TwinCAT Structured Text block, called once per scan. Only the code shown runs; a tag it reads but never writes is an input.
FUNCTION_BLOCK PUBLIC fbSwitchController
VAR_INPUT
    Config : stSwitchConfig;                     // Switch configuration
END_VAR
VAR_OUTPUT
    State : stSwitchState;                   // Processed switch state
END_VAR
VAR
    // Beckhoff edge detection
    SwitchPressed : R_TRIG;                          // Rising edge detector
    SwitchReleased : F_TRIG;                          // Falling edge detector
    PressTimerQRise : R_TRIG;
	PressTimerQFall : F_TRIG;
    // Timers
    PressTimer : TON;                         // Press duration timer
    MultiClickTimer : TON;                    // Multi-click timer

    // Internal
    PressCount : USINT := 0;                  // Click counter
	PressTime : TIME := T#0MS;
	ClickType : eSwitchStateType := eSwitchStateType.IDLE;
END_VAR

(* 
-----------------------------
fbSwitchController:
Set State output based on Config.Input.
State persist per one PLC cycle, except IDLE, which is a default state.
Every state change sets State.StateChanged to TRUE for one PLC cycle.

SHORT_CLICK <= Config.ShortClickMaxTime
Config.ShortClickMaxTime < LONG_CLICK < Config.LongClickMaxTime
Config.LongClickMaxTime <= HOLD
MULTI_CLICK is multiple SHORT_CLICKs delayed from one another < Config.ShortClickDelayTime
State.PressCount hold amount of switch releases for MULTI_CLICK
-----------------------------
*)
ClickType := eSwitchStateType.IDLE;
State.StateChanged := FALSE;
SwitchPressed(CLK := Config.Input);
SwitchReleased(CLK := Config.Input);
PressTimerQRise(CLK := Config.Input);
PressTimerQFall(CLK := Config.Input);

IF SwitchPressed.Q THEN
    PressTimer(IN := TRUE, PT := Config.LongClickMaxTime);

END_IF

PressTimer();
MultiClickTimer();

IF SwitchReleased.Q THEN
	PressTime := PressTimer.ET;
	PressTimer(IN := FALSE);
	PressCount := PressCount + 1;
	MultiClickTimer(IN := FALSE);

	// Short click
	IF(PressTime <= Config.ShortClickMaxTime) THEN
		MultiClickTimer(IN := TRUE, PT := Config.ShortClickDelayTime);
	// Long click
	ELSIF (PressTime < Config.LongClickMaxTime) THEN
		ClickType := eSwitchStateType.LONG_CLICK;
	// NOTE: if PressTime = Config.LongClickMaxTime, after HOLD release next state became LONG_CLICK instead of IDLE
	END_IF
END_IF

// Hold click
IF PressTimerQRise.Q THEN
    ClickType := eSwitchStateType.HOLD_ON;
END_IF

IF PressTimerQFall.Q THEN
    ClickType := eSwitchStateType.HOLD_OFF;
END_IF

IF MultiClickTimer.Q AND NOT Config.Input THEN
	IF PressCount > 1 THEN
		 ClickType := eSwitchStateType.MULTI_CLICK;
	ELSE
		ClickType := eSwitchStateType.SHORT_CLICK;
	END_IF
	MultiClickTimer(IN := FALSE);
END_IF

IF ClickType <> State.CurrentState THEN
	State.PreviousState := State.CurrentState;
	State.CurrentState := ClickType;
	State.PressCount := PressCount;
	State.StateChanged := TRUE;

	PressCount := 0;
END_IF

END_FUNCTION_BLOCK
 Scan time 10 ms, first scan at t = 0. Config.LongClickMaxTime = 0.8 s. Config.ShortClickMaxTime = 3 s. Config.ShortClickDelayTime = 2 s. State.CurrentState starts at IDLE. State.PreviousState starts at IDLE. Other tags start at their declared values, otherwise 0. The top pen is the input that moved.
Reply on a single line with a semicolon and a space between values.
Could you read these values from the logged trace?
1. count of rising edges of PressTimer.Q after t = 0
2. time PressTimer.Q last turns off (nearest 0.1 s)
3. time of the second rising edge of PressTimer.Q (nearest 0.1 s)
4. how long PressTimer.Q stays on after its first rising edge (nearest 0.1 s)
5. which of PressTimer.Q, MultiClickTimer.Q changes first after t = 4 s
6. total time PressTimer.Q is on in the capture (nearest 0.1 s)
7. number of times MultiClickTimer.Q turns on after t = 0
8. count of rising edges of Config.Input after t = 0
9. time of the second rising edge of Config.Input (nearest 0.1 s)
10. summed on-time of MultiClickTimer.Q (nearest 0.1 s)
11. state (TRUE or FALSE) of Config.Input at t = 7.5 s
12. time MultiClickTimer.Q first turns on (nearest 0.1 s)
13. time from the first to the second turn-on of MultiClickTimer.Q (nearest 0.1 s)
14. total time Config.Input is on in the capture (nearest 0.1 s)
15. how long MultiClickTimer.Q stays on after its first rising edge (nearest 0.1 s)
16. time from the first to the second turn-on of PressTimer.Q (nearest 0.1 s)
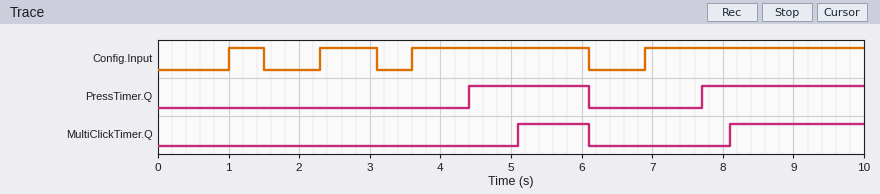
2; 6.1 s; 7.7 s; 1.7 s; PressTimer.Q; 4.0 s; 2; 4; 2.3 s; 2.9 s; TRUE; 5.1 s; 3.0 s; 6.9 s; 1.0 s; 3.3 s
